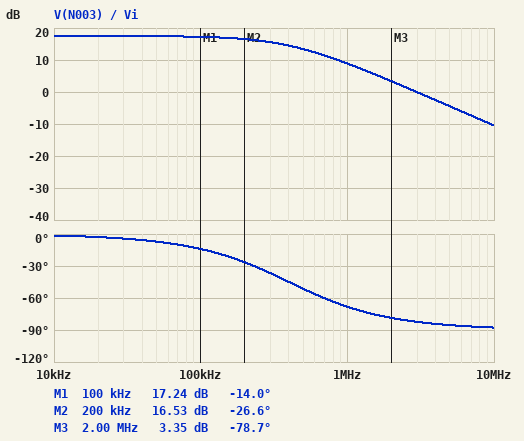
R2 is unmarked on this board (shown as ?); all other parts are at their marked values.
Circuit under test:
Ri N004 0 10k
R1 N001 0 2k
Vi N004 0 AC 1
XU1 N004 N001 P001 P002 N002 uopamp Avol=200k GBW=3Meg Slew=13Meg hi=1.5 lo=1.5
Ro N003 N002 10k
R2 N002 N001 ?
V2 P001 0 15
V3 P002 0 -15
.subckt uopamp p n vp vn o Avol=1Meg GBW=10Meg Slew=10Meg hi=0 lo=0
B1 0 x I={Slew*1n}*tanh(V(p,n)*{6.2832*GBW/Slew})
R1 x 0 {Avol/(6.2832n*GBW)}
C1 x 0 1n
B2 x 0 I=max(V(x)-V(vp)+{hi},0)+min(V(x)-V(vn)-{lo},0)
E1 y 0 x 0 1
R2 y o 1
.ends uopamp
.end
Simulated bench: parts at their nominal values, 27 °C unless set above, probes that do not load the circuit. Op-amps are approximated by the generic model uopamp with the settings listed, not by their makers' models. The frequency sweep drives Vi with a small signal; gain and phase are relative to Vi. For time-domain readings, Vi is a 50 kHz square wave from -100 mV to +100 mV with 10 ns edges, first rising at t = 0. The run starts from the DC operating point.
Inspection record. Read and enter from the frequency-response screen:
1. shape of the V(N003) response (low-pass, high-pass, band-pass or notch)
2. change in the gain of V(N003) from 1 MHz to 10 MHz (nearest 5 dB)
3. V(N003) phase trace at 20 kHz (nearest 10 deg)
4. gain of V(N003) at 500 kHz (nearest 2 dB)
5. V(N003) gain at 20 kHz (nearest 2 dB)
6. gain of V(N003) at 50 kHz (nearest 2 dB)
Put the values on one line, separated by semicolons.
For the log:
low-pass; -20 dB; 0 deg; 14 dB; 18 dB; 18 dB
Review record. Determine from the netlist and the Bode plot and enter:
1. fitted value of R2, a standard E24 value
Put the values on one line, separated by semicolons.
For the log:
13 kΩ
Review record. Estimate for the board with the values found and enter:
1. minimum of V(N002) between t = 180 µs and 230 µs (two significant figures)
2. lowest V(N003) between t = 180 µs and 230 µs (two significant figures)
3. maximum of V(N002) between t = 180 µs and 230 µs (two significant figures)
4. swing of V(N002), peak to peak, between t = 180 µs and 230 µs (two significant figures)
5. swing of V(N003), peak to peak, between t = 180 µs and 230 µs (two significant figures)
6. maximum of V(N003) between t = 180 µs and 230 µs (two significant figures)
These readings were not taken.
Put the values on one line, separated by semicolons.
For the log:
-750 mV; -750 mV; 750 mV; 1.5 V; 1.5 V; 750 mV
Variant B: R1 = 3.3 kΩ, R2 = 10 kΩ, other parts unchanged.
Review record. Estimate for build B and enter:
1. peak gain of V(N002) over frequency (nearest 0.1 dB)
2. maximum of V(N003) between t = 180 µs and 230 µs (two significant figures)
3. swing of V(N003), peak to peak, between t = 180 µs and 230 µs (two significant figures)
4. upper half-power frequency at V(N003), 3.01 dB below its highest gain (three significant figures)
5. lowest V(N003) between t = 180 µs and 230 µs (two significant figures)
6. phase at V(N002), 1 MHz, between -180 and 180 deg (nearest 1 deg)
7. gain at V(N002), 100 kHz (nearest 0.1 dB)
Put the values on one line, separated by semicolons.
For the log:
12.1 dB; 400 mV; 810 mV; 744 kHz; -400 mV; -53 deg; 12.0 dB
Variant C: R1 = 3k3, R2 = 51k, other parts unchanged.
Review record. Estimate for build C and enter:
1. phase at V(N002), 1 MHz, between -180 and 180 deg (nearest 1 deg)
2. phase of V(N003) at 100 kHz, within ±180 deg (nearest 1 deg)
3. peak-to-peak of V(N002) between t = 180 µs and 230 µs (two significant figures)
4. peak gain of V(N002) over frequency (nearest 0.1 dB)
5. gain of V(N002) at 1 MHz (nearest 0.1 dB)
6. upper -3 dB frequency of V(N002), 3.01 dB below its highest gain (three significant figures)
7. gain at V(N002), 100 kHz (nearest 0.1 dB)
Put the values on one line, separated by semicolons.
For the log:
-80 deg; -29 deg; 3.3 V; 24.3 dB; 9.4 dB; 182 kHz; 23.2 dB
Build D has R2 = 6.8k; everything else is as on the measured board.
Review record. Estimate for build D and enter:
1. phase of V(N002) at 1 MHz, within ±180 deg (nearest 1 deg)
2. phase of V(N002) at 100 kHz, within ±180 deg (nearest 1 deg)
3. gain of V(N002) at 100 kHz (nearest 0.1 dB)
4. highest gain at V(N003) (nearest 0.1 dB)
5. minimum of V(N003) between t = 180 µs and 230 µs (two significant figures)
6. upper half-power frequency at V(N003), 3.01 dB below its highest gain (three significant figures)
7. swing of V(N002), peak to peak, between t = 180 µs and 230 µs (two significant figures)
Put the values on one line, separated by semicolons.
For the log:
-56 deg; -8 deg; 12.8 dB; 12.9 dB; -440 mV; 682 kHz; 880 mV
